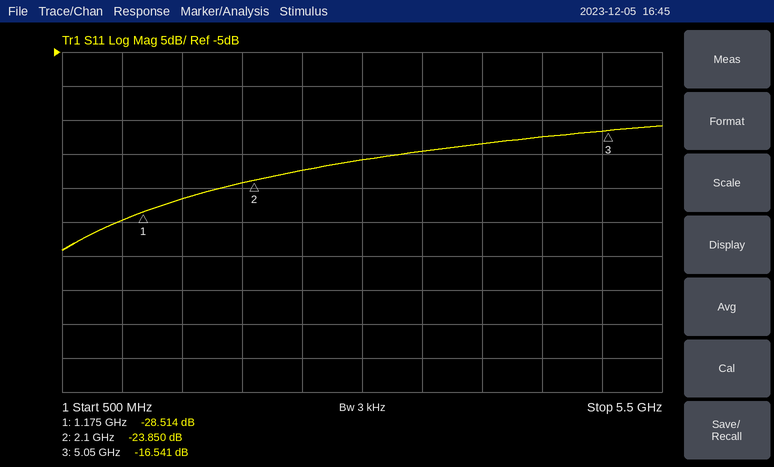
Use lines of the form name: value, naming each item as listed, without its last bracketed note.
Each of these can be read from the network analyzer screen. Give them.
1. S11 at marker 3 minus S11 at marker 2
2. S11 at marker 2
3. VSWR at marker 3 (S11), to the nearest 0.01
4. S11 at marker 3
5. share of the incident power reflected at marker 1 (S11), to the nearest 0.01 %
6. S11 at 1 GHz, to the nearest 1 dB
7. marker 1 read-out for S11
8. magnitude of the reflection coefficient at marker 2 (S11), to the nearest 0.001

S11 at marker 3 minus S11 at marker 2: 7.309 dB
S11 at marker 2: -23.850 dB
VSWR at marker 3 (S11), to the nearest 0.01: 1.35
S11 at marker 3: -16.541 dB
share of the incident power reflected at marker 1 (S11), to the nearest 0.01 %: 0.14 %
S11 at 1 GHz, to the nearest 1 dB: -30 dB
marker 1 read-out for S11: -28.514 dB
magnitude of the reflection coefficient at marker 2 (S11), to the nearest 0.001: 0.064
